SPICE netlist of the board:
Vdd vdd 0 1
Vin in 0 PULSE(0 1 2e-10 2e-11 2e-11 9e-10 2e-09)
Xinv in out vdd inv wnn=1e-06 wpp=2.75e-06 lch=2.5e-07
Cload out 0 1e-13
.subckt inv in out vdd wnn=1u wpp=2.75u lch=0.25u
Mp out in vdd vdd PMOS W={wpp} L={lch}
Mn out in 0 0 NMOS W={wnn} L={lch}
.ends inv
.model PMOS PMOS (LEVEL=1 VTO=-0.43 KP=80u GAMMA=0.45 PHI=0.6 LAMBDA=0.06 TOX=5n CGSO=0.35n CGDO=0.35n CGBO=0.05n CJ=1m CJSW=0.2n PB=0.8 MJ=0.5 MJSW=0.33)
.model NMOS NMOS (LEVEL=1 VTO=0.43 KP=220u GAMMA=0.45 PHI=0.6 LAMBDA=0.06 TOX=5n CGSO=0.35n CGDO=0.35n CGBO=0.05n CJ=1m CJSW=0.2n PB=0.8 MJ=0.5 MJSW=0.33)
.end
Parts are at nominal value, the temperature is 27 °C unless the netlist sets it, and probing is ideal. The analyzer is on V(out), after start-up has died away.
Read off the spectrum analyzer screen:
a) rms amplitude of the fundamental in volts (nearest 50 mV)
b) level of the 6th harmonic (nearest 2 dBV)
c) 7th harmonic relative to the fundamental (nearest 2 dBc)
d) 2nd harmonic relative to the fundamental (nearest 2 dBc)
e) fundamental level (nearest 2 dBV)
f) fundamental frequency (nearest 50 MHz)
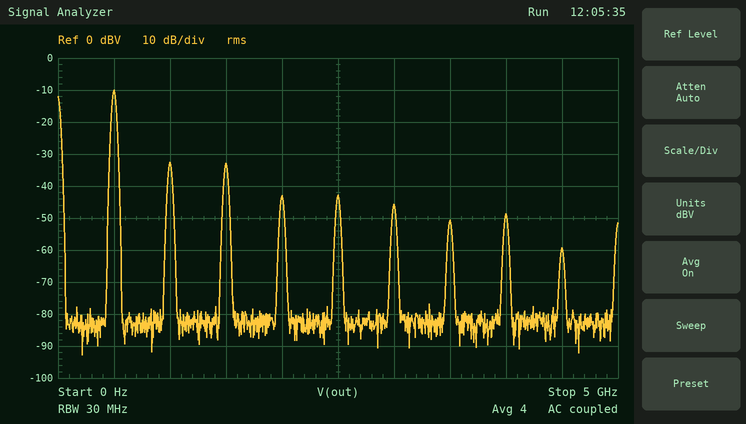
300 mV
-46 dBV
-40 dBc
-22 dBc
-10 dBV
500 MHz
